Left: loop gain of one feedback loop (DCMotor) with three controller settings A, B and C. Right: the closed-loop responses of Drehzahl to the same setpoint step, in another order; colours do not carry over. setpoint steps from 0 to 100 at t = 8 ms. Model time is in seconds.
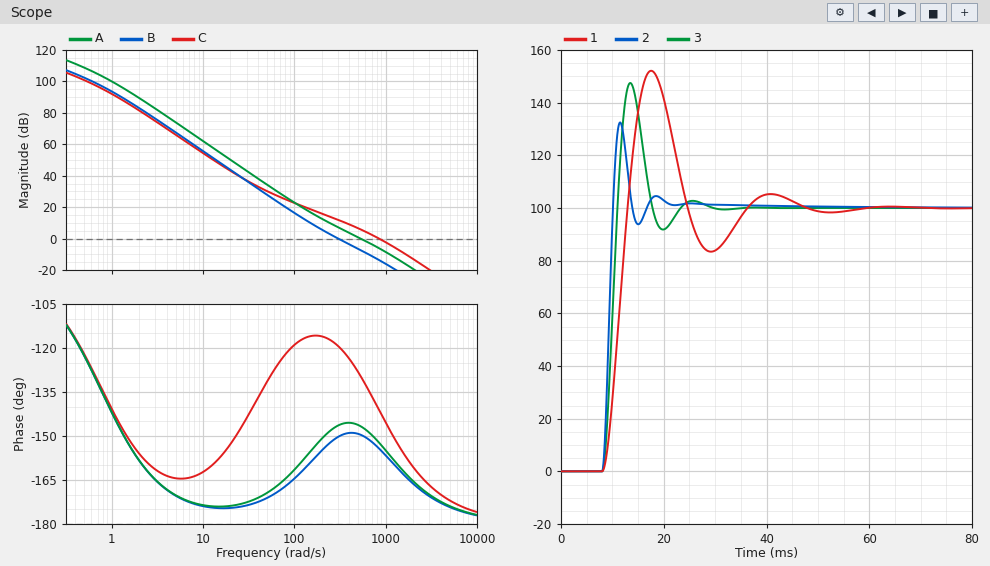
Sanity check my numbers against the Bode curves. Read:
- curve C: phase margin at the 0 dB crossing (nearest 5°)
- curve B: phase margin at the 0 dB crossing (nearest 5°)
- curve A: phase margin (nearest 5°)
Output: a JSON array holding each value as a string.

["40°", "30°", "35°"]
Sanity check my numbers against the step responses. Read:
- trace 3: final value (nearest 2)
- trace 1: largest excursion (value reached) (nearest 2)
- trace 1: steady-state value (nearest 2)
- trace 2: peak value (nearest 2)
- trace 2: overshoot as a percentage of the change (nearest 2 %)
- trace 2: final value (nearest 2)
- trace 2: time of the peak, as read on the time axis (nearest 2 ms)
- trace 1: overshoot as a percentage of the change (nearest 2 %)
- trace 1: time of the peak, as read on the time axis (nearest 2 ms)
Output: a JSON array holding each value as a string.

["100", "152", "100", "132", "32 %", "100", "12 ms", "52 %", "18 ms"]
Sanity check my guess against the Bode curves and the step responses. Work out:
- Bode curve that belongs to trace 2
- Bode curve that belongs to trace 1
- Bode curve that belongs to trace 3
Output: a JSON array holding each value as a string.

["C", "B", "A"]
